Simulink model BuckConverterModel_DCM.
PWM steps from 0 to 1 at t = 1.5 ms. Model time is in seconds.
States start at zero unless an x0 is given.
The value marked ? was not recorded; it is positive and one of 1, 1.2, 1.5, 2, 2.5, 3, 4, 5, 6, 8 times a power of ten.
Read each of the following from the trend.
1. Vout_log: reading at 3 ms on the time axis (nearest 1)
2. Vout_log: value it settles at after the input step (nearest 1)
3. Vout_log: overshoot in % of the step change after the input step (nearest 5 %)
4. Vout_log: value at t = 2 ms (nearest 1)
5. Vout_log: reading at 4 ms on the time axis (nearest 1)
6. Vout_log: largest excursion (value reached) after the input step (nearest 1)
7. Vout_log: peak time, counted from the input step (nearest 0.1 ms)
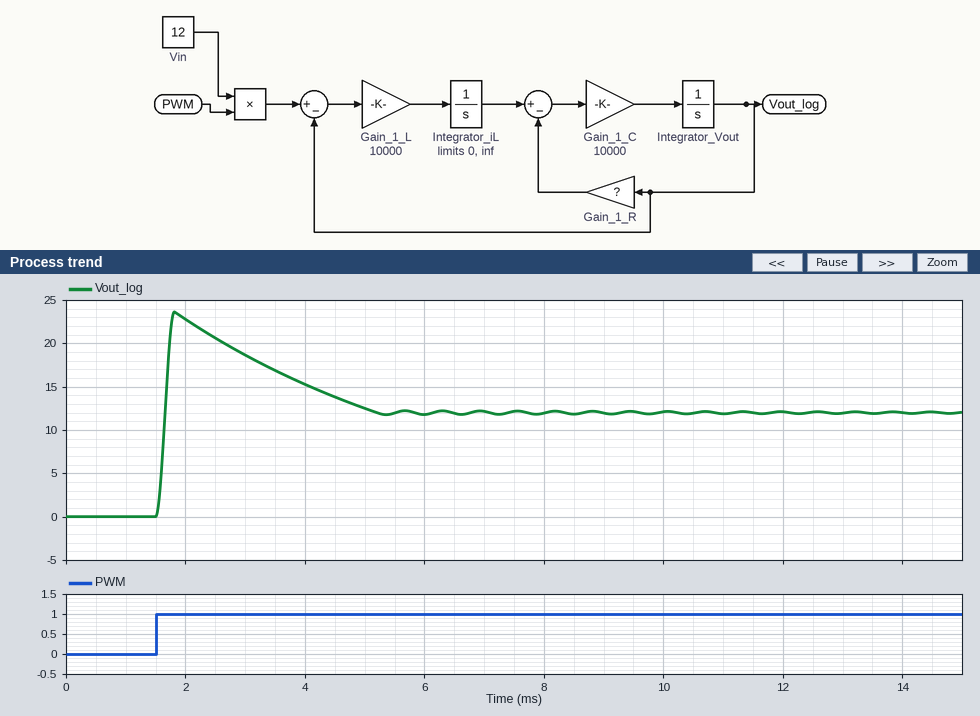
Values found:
19
12
95 %
23
15
24
0.3 ms
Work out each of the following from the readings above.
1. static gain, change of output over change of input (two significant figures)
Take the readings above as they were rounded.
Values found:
12
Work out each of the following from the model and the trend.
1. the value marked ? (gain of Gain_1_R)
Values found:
0.02
